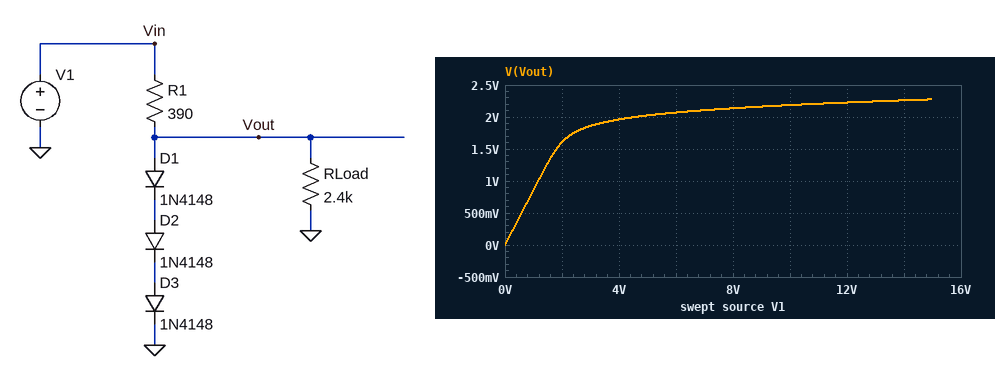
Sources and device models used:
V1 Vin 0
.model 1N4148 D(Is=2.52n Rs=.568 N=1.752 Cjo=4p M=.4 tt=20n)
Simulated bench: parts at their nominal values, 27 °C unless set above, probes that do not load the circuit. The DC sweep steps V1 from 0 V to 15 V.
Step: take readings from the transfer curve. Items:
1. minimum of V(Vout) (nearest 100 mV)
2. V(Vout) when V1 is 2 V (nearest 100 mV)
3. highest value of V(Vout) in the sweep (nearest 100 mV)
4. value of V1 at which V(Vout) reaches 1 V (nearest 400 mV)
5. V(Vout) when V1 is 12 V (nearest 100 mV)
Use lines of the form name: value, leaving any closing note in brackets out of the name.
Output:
minimum of V(Vout): 0 V
V(Vout) when V1 is 2 V: 1.6 V
highest value of V(Vout) in the sweep: 2.3 V
value of V1 at which V(Vout) reaches 1 V: 1.2 V
V(Vout) when V1 is 12 V: 2.2 V
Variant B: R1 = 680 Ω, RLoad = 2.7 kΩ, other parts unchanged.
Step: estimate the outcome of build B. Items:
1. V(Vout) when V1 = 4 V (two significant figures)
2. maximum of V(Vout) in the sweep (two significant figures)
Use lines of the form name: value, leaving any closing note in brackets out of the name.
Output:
V(Vout) when V1 = 4 V: 1.9 V
maximum of V(Vout) in the sweep: 2.2 V
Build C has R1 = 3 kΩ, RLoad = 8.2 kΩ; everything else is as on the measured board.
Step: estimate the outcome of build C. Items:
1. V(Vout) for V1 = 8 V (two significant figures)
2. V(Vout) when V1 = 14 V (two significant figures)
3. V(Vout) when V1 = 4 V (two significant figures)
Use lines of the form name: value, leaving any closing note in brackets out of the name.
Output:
V(Vout) for V1 = 8 V: 1.8 V
V(Vout) when V1 = 14 V: 1.9 V
V(Vout) when V1 = 4 V: 1.7 V
